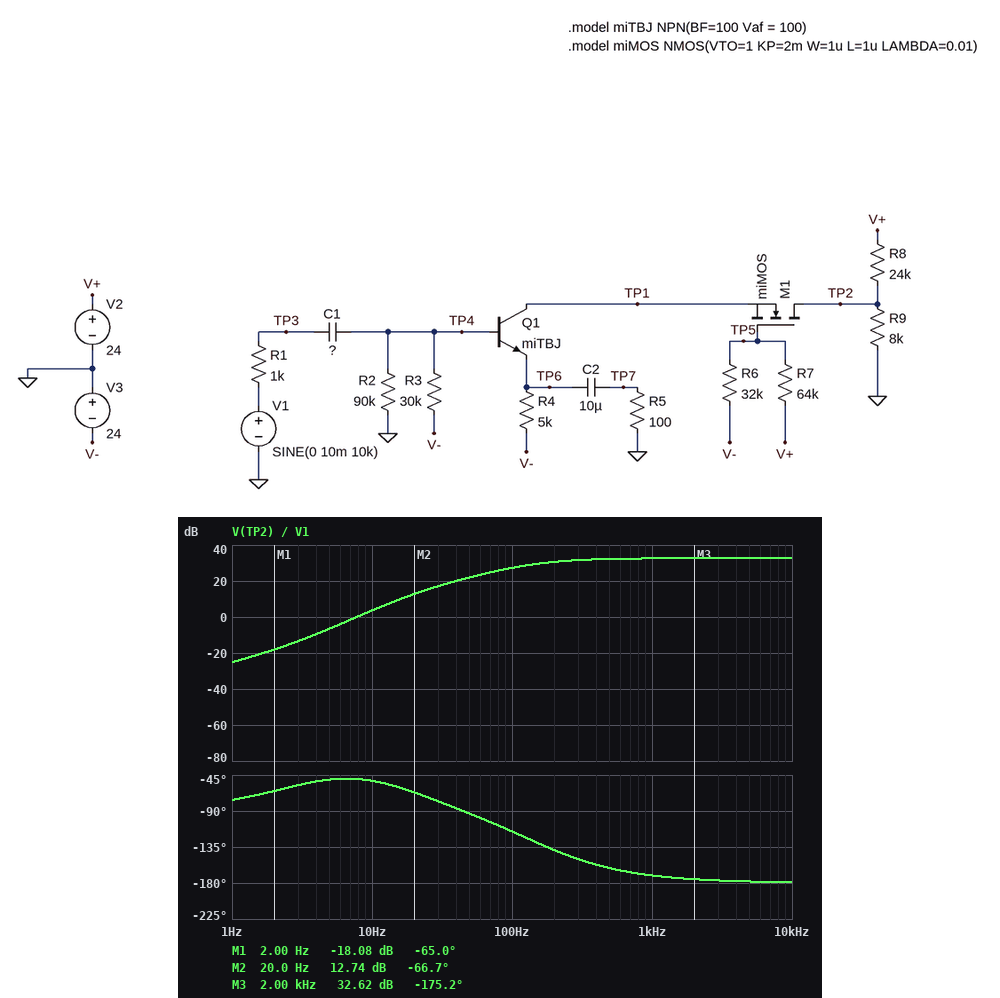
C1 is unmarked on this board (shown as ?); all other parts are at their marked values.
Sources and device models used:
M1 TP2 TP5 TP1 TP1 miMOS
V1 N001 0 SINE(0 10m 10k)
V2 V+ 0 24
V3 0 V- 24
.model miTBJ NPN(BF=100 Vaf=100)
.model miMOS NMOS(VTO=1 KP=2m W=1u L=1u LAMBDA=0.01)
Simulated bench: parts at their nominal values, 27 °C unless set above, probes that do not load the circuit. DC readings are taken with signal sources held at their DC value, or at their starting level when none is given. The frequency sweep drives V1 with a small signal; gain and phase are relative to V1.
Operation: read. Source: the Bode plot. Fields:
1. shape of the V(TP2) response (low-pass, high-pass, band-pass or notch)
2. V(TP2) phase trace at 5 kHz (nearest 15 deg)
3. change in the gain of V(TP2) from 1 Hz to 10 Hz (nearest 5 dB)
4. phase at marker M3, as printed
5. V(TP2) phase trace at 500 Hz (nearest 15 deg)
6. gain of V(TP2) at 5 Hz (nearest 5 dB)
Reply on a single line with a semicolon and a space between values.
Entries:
high-pass; -180 deg; 30 dB; -175.2 deg; -165 deg; -5 dB
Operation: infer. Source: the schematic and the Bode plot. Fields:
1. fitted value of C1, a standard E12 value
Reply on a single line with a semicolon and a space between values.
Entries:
330 nF
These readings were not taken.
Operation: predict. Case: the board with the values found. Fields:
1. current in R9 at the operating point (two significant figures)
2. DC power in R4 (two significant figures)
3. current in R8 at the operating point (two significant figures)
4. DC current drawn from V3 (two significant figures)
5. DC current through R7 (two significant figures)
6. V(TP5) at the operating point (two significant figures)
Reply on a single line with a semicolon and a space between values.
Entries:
3.7 µA; 5.0 mW; 1.0 mA; 1.7 mA; 500 µA; -8.0 V
